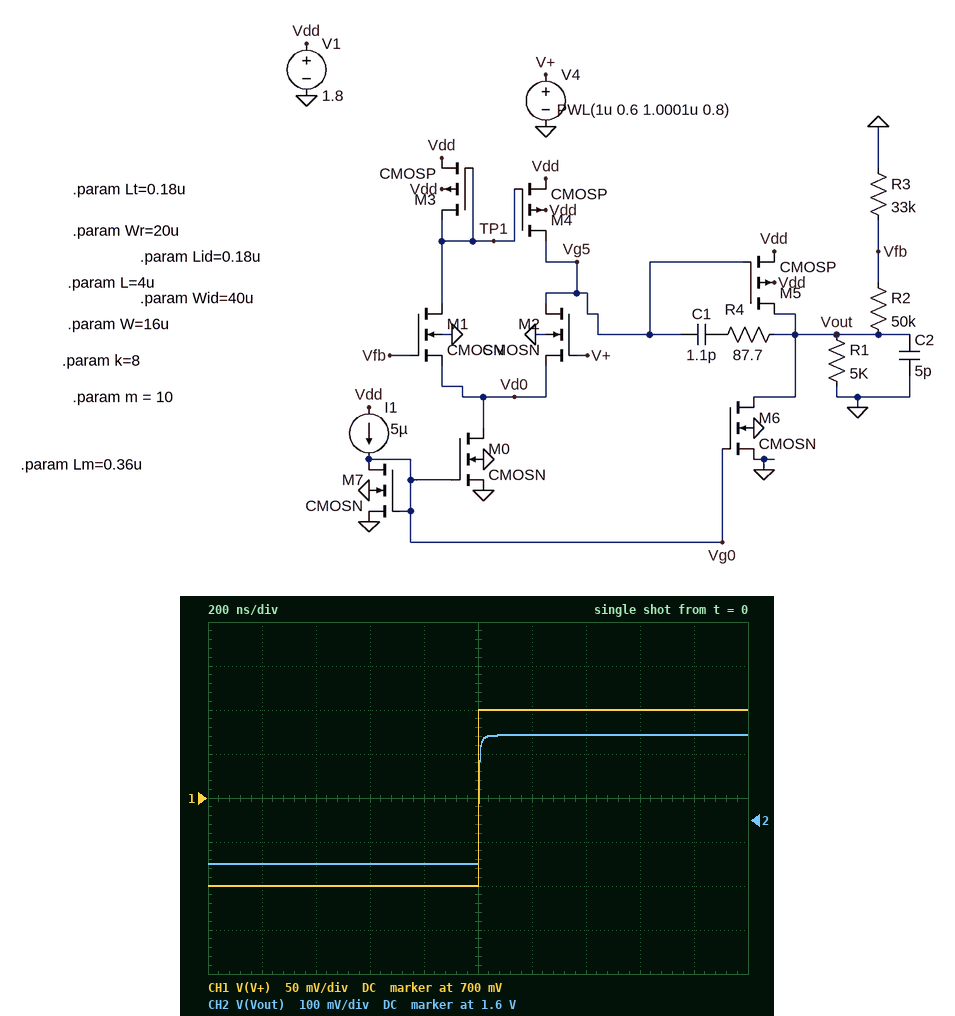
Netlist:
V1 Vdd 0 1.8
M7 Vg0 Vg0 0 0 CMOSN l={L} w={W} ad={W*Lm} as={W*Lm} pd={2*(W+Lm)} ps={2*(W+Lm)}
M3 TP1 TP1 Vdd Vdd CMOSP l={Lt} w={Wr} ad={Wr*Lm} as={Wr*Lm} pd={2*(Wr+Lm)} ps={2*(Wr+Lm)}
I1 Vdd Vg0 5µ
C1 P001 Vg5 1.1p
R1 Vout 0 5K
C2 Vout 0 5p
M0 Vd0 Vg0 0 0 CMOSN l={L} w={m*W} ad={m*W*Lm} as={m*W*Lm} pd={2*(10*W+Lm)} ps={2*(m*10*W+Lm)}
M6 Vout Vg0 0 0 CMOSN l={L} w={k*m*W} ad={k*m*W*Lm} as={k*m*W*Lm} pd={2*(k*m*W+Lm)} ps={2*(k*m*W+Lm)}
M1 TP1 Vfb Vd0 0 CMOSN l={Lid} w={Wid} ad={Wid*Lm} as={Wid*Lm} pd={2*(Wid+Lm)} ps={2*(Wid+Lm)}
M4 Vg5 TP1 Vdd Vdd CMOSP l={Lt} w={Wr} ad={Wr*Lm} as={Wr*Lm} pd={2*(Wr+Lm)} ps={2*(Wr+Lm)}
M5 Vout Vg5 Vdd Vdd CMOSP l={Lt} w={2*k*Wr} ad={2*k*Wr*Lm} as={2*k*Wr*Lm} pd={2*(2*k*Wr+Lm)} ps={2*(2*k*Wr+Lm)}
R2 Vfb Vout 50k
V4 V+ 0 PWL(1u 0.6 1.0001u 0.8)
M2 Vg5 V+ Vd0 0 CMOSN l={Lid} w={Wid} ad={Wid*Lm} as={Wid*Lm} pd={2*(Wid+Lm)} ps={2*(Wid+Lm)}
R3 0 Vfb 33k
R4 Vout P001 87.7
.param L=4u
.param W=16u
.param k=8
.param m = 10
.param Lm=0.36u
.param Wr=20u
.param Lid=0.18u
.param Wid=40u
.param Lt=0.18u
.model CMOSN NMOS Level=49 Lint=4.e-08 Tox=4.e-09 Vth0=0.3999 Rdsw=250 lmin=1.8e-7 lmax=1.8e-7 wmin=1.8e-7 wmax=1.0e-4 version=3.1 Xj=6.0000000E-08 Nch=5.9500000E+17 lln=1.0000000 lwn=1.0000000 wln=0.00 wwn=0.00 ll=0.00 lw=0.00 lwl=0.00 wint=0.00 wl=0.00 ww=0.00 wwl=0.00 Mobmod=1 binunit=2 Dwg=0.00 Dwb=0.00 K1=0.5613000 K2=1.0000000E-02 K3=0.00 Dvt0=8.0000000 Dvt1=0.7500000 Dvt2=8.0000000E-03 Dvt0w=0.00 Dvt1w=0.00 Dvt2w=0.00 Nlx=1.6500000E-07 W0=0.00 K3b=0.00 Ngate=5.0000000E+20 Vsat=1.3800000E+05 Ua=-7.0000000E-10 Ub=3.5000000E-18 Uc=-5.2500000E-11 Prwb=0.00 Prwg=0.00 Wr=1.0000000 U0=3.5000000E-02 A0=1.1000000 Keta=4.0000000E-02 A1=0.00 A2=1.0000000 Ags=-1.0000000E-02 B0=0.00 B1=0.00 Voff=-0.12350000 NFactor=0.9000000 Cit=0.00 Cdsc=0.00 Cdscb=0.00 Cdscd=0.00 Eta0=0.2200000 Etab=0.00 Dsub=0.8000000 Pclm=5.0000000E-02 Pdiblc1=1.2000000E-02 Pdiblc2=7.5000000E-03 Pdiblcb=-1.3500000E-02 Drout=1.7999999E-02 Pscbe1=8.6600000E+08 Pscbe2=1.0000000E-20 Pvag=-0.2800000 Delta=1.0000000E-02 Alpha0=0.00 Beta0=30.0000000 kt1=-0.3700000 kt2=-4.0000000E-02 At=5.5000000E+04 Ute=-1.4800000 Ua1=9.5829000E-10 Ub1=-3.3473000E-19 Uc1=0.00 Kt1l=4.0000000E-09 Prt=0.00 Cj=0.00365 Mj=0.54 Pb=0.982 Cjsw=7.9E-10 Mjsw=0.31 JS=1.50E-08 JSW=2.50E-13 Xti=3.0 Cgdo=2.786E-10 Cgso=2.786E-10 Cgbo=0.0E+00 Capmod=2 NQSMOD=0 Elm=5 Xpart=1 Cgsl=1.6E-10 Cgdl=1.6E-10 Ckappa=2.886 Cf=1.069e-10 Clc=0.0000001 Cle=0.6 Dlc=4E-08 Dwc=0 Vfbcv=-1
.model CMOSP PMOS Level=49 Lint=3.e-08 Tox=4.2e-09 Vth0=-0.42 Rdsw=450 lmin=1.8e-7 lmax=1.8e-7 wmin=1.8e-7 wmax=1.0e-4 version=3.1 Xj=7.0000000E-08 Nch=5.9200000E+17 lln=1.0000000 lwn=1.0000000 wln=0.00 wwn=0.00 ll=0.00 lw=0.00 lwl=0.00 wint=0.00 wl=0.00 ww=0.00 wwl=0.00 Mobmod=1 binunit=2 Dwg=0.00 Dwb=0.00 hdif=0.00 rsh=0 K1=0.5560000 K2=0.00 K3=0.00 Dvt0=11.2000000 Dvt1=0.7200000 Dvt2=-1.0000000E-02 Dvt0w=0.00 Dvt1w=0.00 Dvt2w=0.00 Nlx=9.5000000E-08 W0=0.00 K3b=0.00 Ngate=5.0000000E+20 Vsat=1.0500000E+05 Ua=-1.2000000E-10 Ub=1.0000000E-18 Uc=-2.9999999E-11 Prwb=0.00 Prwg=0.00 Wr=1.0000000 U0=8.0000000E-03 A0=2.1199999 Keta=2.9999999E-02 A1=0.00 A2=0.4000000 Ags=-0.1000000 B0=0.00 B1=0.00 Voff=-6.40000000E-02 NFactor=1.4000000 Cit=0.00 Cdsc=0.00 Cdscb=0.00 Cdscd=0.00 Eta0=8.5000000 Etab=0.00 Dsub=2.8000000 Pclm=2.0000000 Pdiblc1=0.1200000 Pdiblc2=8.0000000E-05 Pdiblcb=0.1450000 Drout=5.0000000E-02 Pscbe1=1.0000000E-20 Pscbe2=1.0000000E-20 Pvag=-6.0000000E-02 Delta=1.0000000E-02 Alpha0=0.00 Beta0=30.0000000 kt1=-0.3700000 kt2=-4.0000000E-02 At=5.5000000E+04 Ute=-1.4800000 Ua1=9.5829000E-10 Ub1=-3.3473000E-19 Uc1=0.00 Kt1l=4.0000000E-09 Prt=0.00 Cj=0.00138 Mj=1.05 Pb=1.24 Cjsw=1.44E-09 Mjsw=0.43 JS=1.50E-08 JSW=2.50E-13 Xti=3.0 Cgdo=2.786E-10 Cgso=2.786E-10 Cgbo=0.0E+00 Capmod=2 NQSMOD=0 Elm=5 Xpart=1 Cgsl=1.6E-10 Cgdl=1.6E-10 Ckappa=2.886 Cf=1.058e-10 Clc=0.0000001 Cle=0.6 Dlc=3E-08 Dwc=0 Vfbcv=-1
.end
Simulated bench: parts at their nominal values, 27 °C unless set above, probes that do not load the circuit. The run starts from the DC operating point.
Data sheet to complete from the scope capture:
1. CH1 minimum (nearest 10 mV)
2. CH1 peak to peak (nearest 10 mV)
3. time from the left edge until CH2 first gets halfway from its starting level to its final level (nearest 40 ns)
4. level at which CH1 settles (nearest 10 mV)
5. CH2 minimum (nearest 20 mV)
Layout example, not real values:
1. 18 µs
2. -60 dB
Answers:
1. 600 mV
2. 200 mV
3. 1.00 µs
4. 800 mV
5. 1.50 V
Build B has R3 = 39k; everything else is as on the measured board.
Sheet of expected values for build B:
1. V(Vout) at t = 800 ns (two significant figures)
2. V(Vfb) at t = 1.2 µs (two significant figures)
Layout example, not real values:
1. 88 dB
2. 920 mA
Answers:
1. 1.4 V
2. 780 mV
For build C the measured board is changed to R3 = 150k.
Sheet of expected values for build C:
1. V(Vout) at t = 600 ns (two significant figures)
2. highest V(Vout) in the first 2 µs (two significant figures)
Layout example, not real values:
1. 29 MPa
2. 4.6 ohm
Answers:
1. 800 mV
2. 1.1 V
